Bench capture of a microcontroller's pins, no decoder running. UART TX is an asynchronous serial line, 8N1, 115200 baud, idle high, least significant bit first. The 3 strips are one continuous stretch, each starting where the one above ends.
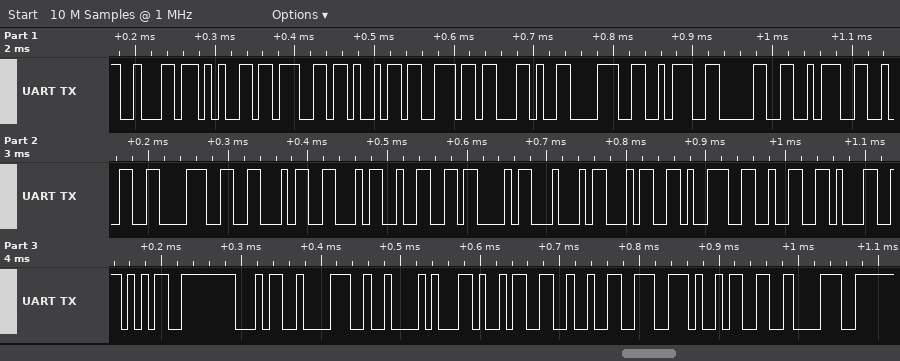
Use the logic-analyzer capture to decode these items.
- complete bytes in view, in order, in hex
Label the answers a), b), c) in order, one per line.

a) 62 65 67 69 6E 2C 38 3A 30 3A 32 38 46 46 32 43 44 34 39 32 31 35 34 38 42 2C 33 32 2E 33 38
